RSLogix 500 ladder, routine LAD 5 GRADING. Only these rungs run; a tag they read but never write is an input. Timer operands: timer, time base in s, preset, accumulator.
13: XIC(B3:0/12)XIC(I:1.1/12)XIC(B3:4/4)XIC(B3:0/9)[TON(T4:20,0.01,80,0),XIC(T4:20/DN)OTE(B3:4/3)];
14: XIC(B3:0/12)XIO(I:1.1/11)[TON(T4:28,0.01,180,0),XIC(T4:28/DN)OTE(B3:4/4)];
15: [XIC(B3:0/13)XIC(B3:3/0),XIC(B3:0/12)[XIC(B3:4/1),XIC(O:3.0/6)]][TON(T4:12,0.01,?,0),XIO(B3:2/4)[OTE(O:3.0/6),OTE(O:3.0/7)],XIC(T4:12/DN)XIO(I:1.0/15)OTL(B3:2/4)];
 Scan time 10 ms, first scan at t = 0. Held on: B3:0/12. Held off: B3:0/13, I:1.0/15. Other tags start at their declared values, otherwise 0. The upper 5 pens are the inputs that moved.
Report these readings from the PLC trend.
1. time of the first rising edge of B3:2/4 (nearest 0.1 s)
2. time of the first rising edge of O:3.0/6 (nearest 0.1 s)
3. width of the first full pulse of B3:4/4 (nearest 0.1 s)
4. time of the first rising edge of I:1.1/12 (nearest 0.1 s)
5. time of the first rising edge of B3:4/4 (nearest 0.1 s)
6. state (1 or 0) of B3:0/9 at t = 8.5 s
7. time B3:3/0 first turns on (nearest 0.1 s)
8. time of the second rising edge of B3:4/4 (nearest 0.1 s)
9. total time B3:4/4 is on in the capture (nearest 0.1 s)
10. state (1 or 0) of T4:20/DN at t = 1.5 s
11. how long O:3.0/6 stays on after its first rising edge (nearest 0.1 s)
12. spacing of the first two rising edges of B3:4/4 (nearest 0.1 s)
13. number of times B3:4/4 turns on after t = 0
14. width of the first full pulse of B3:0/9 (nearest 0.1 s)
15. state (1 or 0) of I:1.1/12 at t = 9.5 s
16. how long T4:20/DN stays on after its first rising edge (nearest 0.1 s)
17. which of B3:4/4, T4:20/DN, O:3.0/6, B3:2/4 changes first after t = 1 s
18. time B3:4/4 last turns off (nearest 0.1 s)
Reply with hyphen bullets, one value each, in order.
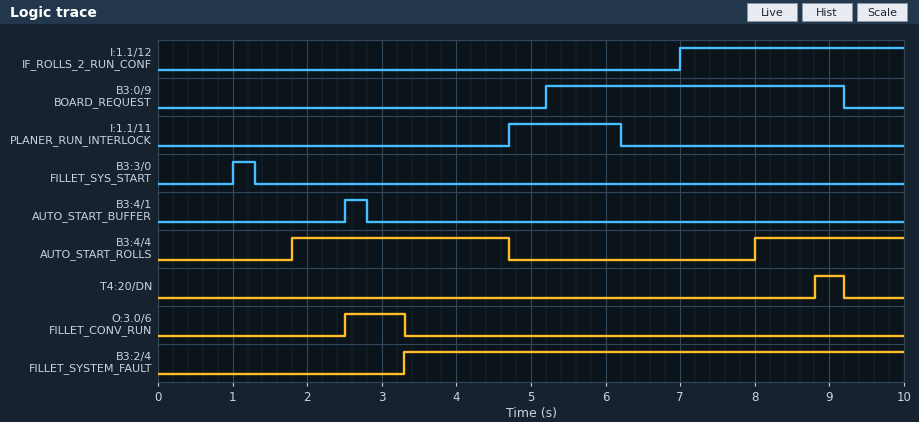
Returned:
- 3.3 s
- 2.5 s
- 2.9 s
- 7.0 s
- 1.8 s
- 1
- 1.0 s
- 8.0 s
- 4.9 s
- 0
- 0.8 s
- 6.2 s
- 2
- 4.0 s
- 1
- 0.4 s
- B3:4/4
- 4.7 s
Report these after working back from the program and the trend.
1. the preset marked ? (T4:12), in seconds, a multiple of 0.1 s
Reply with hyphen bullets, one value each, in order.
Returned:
- 0.8 s
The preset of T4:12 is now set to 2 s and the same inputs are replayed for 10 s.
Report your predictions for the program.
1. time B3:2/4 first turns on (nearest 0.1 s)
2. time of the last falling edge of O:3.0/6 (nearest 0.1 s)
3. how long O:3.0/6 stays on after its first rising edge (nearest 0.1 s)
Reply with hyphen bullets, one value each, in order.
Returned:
- 4.5 s
- 4.5 s
- 2.0 s
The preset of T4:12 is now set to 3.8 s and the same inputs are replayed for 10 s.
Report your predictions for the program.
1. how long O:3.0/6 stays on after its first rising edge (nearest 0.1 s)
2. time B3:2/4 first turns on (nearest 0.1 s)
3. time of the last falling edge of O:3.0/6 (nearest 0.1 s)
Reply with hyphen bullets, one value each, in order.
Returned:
- 3.8 s
- 6.3 s
- 6.3 s
